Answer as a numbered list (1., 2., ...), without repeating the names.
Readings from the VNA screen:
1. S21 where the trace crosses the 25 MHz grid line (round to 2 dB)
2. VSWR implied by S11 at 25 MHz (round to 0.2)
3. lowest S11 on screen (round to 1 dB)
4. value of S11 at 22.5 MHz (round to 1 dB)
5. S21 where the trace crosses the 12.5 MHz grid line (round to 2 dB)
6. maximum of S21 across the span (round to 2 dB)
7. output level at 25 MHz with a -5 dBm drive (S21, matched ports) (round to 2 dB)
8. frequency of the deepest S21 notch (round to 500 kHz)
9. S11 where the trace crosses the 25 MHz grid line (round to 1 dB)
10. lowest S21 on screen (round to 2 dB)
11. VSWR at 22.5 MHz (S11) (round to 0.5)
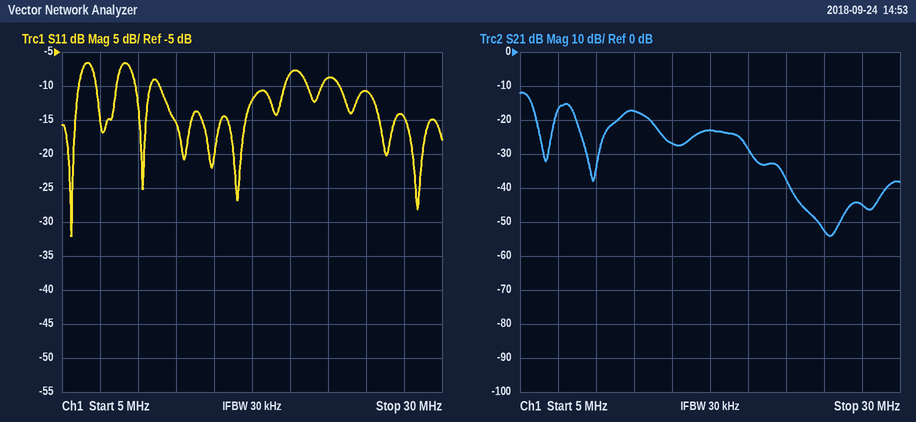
1. -52 dB
2. 1.8
3. -32 dB
4. -9 dB
5. -18 dB
6. -12 dB
7. -58 dBm
8. 25.5 MHz
9. -11 dB
10. -54 dB
11. 2.0
